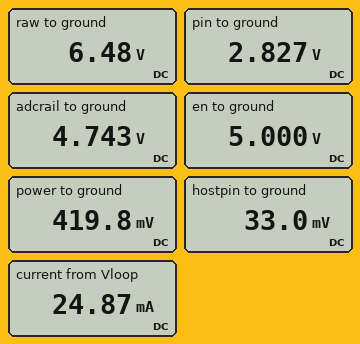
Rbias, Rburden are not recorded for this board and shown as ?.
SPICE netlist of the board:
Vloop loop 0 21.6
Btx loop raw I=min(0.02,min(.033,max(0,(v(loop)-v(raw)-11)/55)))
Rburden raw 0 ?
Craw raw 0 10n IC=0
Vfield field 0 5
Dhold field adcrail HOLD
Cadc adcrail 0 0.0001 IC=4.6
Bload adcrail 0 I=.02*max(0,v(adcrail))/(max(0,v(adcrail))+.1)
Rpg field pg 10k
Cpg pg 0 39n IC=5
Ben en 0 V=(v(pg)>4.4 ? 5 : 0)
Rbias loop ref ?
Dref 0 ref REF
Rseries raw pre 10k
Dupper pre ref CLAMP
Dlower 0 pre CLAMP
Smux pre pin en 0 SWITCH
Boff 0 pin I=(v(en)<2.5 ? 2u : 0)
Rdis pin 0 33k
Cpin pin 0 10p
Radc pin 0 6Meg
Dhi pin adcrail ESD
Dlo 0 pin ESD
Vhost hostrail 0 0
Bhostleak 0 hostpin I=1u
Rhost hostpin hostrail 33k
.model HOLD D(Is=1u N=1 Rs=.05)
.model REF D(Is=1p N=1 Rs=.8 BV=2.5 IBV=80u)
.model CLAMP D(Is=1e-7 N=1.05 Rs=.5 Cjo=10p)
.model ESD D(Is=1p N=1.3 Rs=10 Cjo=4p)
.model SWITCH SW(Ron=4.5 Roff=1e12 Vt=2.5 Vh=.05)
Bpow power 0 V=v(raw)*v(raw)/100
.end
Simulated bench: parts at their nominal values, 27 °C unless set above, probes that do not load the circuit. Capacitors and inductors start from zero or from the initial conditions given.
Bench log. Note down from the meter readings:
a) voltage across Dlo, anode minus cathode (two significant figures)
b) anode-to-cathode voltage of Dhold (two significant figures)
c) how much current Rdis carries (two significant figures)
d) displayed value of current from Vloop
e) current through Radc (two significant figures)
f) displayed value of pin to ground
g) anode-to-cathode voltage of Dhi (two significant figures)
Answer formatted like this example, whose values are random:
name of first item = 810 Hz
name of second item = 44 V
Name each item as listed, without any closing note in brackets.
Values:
voltage across Dlo, anode minus cathode = -2.8 V
anode-to-cathode voltage of Dhold = 260 mV
how much current Rdis carries = 86 µA
displayed value of current from Vloop = 24.87 mA
current through Radc = 470 nA
displayed value of pin to ground = 2.827 V
anode-to-cathode voltage of Dhi = -1.9 V
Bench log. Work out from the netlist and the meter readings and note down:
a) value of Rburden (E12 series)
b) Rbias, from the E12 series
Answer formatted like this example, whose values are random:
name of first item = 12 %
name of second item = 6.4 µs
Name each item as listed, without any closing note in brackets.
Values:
value of Rburden = 330 Ω
Rbias, from the E12 series = 3.9 kΩ
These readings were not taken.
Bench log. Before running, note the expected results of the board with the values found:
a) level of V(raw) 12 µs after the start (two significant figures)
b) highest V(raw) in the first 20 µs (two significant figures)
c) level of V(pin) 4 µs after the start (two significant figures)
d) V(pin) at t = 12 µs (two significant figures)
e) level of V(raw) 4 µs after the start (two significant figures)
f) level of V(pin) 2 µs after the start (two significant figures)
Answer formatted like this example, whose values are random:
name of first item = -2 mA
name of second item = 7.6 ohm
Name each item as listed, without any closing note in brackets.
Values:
level of V(raw) 12 µs after the start = 6.3 V
highest V(raw) in the first 20 µs = 6.5 V
level of V(pin) 4 µs after the start = 2.8 V
V(pin) at t = 12 µs = 2.8 V
level of V(raw) 4 µs after the start = 4.6 V
level of V(pin) 2 µs after the start = 2.1 V
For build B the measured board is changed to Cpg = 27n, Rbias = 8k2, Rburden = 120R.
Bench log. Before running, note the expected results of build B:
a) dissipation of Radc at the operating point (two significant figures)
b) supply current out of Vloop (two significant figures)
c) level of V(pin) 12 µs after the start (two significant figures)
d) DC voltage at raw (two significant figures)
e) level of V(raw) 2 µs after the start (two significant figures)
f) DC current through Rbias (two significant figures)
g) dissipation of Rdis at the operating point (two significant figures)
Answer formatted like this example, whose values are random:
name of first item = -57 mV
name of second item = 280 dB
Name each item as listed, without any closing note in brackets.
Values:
dissipation of Radc at the operating point = 560 nW
supply current out of Vloop = 22 mA
level of V(pin) 12 µs after the start = 1.8 V
DC voltage at raw = 2.4 V
level of V(raw) 2 µs after the start = 1.9 V
DC current through Rbias = 2.3 mA
dissipation of Rdis at the operating point = 100 µW
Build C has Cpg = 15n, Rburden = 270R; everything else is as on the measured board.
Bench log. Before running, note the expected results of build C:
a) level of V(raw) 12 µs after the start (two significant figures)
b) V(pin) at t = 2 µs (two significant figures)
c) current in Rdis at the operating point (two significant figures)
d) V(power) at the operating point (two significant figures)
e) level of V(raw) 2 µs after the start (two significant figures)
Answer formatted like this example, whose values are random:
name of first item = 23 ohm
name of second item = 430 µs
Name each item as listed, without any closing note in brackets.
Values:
level of V(raw) 12 µs after the start = 5.3 V
V(pin) at t = 2 µs = 2.0 V
current in Rdis at the operating point = 85 µA
V(power) at the operating point = 280 mV
level of V(raw) 2 µs after the start = 2.8 V
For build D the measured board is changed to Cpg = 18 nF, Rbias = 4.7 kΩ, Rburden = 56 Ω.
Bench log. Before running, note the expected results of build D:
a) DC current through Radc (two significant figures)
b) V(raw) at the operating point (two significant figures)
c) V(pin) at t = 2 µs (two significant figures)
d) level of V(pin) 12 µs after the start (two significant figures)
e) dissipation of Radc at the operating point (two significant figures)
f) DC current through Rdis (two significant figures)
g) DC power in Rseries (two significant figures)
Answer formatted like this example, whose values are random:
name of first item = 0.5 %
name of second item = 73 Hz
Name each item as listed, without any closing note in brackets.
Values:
DC current through Radc = 140 nA
V(raw) at the operating point = 1.1 V
V(pin) at t = 2 µs = 820 mV
level of V(pin) 12 µs after the start = 860 mV
dissipation of Radc at the operating point = 120 nW
DC current through Rdis = 26 µA
DC power in Rseries = 6.8 µW
